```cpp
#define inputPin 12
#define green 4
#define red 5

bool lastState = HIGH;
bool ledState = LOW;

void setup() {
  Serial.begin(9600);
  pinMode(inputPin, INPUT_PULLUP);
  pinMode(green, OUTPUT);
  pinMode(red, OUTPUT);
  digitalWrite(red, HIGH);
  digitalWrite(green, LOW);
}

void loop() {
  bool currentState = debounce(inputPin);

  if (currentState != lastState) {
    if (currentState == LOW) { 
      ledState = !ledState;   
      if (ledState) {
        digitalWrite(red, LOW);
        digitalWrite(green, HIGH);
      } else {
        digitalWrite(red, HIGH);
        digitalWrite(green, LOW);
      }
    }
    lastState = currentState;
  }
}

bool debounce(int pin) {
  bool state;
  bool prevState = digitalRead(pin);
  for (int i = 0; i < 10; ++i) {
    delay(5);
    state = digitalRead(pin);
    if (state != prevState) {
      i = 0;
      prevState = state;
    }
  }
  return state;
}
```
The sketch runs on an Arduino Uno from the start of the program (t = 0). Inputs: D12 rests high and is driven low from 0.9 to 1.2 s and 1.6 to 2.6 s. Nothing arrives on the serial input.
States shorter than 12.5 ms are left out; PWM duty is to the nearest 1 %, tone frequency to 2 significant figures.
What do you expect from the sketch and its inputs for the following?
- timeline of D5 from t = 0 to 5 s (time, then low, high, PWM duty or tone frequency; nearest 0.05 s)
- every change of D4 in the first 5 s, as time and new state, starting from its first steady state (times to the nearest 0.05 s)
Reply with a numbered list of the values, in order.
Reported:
1. 0 s high; 0.95 s low; 1.65 s high
2. 0 s low; 0.95 s high; 1.65 s low
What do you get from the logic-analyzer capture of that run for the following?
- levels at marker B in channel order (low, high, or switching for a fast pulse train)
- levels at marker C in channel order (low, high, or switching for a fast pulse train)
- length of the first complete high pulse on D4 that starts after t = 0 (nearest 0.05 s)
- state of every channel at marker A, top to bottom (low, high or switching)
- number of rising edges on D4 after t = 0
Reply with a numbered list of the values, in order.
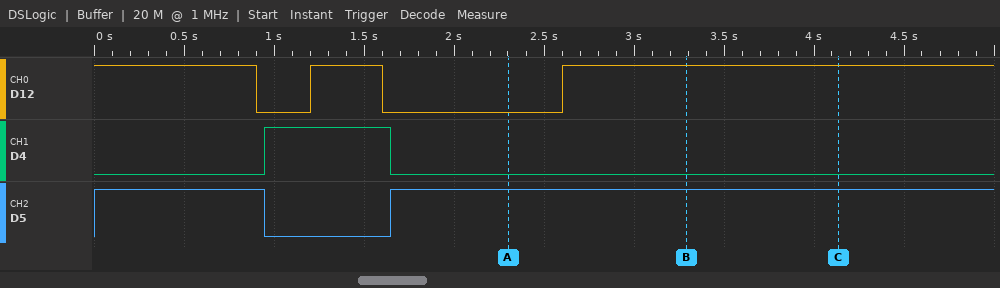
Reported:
1. D12 high, D4 low, D5 high
2. D12 high, D4 low, D5 high
3. 0.70 s
4. D12 low, D4 low, D5 high
5. 1
